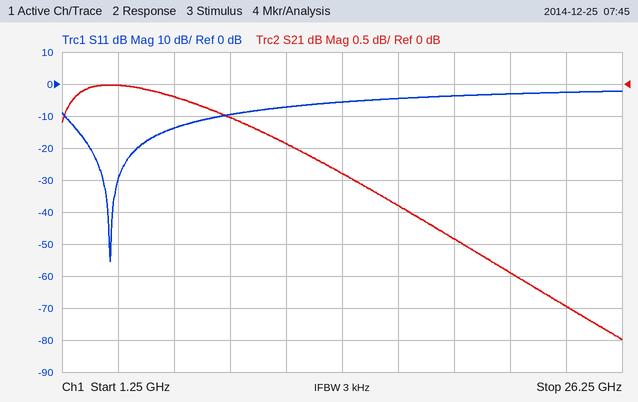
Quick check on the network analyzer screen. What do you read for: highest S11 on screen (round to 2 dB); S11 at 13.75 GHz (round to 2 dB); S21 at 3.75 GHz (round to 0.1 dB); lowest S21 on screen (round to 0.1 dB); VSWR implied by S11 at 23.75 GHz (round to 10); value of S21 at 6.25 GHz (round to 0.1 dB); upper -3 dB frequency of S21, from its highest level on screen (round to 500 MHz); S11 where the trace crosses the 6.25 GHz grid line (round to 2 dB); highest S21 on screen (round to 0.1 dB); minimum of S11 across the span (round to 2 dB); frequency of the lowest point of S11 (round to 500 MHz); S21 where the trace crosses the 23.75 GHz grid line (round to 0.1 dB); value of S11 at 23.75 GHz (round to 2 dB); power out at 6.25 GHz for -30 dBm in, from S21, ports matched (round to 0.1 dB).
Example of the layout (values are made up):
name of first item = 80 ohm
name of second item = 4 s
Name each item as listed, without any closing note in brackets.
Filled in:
highest S11 on screen = -2 dB
S11 at 13.75 GHz = -6 dB
S21 at 3.75 GHz = 0.0 dB
lowest S21 on screen = -4.0 dB
VSWR implied by S11 at 23.75 GHz = 10
value of S21 at 6.25 GHz = -0.2 dB
upper -3 dB frequency of S21, from its highest level on screen = 21.5 GHz
S11 where the trace crosses the 6.25 GHz grid line = -14 dB
highest S21 on screen = 0.0 dB
minimum of S11 across the span = -56 dB
frequency of the lowest point of S11 = 3.5 GHz
S21 where the trace crosses the 23.75 GHz grid line = -3.5 dB
value of S11 at 23.75 GHz = -2 dB
power out at 6.25 GHz for -30 dBm in, from S21, ports matched = -30.2 dBm
